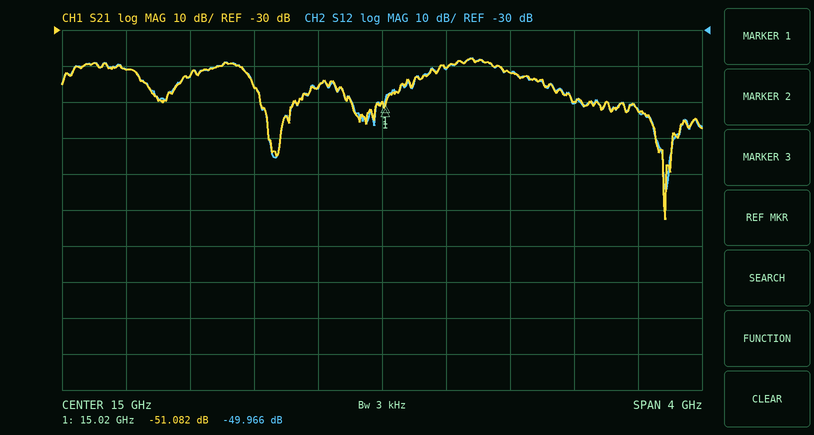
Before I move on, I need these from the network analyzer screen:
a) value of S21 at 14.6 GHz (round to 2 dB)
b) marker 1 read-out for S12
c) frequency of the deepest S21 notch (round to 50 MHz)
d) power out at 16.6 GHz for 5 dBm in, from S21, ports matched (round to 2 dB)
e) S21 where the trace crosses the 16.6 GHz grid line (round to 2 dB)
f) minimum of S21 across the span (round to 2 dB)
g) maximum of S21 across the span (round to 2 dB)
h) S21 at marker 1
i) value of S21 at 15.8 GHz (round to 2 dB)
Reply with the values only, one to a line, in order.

-46 dB
-49.966 dB
16.75 GHz
-48 dBm
-52 dB
-82 dB
-38 dB
-51.082 dB
-42 dB
